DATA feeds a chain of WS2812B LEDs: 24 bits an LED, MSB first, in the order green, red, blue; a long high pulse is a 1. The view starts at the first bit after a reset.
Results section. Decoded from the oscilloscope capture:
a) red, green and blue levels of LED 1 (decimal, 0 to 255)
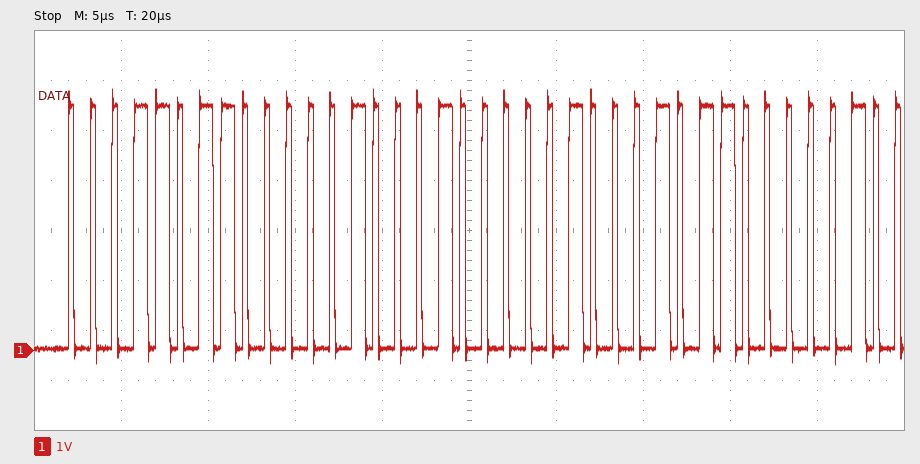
4, 27, 65
